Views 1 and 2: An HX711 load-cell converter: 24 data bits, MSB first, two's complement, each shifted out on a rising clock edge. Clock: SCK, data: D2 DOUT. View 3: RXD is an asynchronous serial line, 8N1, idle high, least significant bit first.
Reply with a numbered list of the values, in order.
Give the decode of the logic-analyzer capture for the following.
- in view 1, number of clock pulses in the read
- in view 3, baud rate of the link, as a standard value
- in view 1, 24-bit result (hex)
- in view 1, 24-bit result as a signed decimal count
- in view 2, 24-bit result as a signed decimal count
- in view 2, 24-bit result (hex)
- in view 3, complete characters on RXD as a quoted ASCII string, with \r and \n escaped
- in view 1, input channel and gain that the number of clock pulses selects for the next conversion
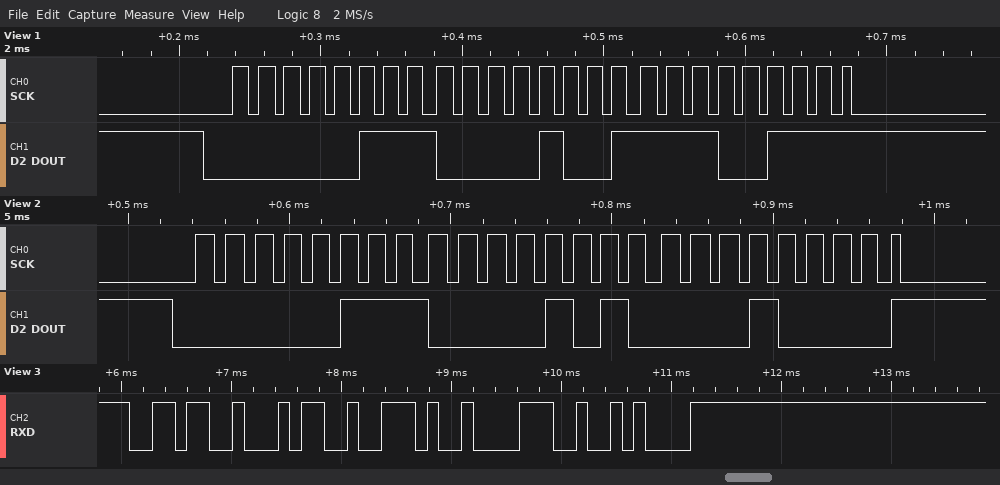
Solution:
1. 25
2. 9600 baud
3. 0x0709E7
4. 461287
5. 461328
6. 0x070A10
7. "64.8\n"
8. channel A, gain 128
